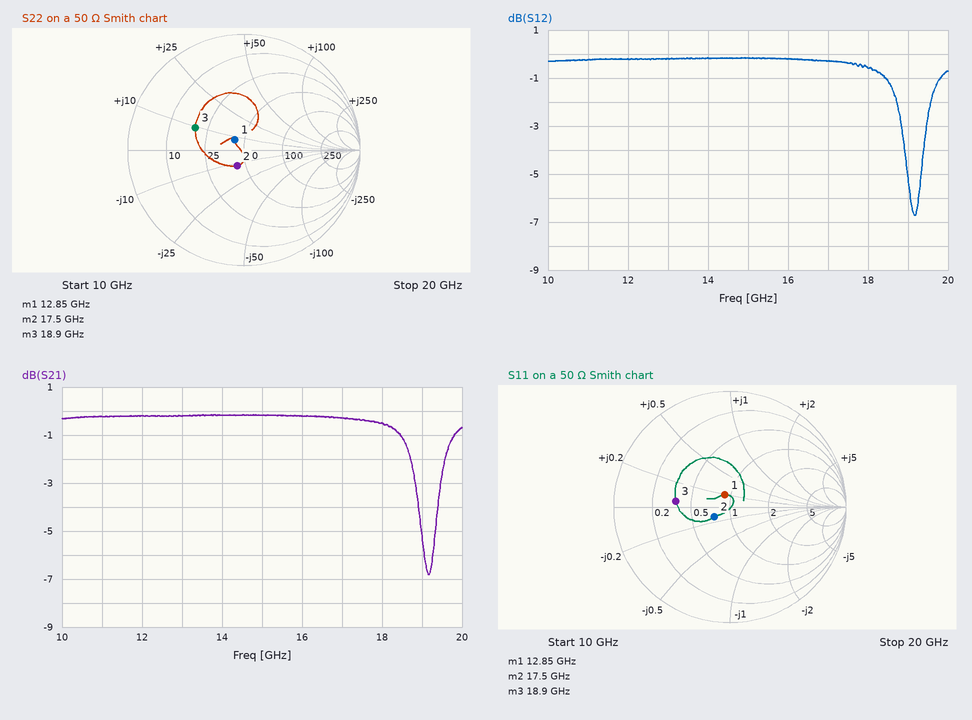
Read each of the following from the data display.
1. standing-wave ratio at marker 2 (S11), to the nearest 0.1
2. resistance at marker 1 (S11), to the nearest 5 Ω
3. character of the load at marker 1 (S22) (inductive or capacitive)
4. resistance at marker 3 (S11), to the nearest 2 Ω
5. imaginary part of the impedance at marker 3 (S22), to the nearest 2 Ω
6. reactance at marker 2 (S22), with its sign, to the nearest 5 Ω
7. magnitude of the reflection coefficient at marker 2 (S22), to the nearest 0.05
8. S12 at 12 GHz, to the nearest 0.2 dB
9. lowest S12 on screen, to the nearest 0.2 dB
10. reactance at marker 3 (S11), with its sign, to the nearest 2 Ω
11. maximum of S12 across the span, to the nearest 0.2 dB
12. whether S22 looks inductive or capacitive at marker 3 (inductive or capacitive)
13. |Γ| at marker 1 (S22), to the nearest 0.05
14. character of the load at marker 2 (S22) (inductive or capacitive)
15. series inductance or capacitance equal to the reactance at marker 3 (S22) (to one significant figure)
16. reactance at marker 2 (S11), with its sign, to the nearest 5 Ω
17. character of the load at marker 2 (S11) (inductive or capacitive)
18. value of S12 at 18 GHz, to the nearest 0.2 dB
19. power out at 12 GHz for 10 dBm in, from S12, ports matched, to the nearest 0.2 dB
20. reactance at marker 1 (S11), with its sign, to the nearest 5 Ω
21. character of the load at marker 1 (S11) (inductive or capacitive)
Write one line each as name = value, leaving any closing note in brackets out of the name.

standing-wave ratio at marker 2 (S11), to the nearest 0.1 = 1.4
resistance at marker 1 (S11), to the nearest 5 Ω = 45 Ω
character of the load at marker 1 (S22) = inductive
resistance at marker 3 (S11), to the nearest 2 Ω = 18 Ω
imaginary part of the impedance at marker 3 (S22), to the nearest 2 Ω = +10 Ω
reactance at marker 2 (S22), with its sign, to the nearest 5 Ω = -10 Ω
magnitude of the reflection coefficient at marker 2 (S22), to the nearest 0.05 = 0.15
S12 at 12 GHz, to the nearest 0.2 dB = -0.2 dB
lowest S12 on screen, to the nearest 0.2 dB = -6.8 dB
reactance at marker 3 (S11), with its sign, to the nearest 2 Ω = +2 Ω
maximum of S12 across the span, to the nearest 0.2 dB = -0.2 dB
whether S22 looks inductive or capacitive at marker 3 = inductive
|Γ| at marker 1 (S22), to the nearest 0.05 = 0.10
character of the load at marker 2 (S22) = capacitive
series inductance or capacitance equal to the reactance at marker 3 (S22) = 80 pH
reactance at marker 2 (S11), with its sign, to the nearest 5 Ω = -5 Ω
character of the load at marker 2 (S11) = capacitive
value of S12 at 18 GHz, to the nearest 0.2 dB = -0.6 dB
power out at 12 GHz for 10 dBm in, from S12, ports matched, to the nearest 0.2 dB = 9.8 dBm
reactance at marker 1 (S11), with its sign, to the nearest 5 Ω = +10 Ω
character of the load at marker 1 (S11) = inductive
